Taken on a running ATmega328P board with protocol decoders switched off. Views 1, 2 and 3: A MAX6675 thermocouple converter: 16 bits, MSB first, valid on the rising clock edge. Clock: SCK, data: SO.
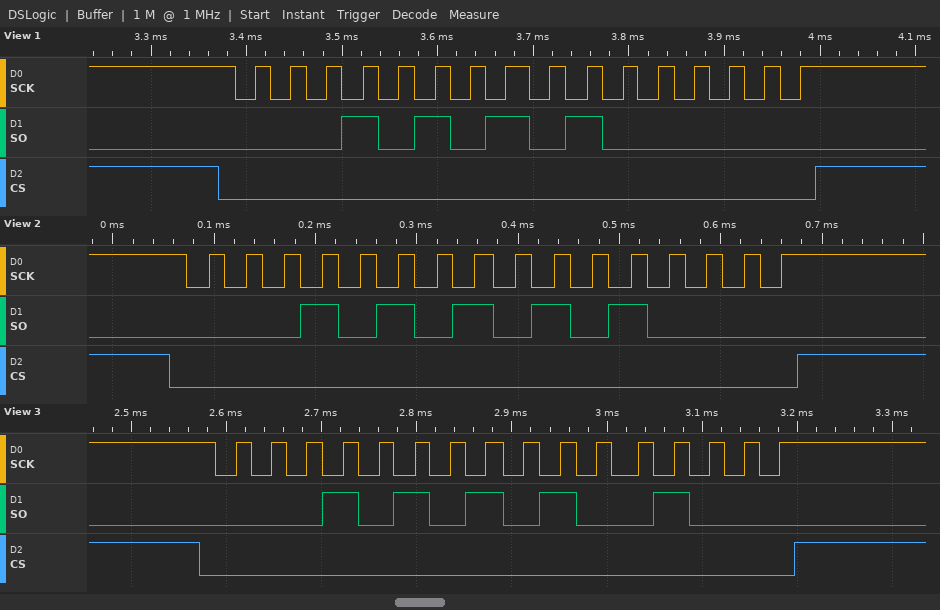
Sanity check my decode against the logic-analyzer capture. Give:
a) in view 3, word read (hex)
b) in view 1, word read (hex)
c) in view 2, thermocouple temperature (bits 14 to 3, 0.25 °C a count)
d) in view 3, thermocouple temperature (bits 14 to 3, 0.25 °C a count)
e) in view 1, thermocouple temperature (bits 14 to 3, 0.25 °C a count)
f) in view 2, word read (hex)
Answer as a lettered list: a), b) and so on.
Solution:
a) 0x1548
b) 0x1540
c) 170.50 °C
d) 170.25 °C
e) 170.00 °C
f) 0x1550
